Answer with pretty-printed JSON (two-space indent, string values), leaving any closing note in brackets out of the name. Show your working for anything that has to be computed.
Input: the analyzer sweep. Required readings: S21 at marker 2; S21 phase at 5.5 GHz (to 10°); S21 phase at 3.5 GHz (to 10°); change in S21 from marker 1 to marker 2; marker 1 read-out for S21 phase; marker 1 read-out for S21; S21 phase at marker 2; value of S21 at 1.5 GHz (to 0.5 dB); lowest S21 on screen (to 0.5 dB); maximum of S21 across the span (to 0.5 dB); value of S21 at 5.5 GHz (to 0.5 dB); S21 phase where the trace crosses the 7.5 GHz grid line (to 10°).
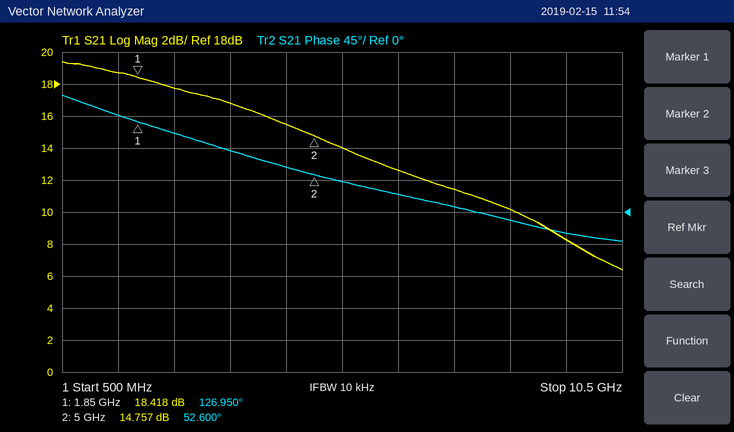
{
  "S21 at marker 2": "14.757 dB",
  "S21 phase at 5.5 GHz": "40°",
  "S21 phase at 3.5 GHz": "90°",
  "change in S21 from marker 1 to marker 2": "14.757 − (18.418) = -3.661 dB",
  "marker 1 read-out for S21 phase": "126.950°",
  "marker 1 read-out for S21": "18.418 dB",
  "S21 phase at marker 2": "52.600°",
  "value of S21 at 1.5 GHz": "18.5 dB",
  "lowest S21 on screen": "6.5 dB",
  "maximum of S21 across the span": "19.5 dB",
  "value of S21 at 5.5 GHz": "14.0 dB",
  "S21 phase where the trace crosses the 7.5 GHz grid line": "10°"
}
